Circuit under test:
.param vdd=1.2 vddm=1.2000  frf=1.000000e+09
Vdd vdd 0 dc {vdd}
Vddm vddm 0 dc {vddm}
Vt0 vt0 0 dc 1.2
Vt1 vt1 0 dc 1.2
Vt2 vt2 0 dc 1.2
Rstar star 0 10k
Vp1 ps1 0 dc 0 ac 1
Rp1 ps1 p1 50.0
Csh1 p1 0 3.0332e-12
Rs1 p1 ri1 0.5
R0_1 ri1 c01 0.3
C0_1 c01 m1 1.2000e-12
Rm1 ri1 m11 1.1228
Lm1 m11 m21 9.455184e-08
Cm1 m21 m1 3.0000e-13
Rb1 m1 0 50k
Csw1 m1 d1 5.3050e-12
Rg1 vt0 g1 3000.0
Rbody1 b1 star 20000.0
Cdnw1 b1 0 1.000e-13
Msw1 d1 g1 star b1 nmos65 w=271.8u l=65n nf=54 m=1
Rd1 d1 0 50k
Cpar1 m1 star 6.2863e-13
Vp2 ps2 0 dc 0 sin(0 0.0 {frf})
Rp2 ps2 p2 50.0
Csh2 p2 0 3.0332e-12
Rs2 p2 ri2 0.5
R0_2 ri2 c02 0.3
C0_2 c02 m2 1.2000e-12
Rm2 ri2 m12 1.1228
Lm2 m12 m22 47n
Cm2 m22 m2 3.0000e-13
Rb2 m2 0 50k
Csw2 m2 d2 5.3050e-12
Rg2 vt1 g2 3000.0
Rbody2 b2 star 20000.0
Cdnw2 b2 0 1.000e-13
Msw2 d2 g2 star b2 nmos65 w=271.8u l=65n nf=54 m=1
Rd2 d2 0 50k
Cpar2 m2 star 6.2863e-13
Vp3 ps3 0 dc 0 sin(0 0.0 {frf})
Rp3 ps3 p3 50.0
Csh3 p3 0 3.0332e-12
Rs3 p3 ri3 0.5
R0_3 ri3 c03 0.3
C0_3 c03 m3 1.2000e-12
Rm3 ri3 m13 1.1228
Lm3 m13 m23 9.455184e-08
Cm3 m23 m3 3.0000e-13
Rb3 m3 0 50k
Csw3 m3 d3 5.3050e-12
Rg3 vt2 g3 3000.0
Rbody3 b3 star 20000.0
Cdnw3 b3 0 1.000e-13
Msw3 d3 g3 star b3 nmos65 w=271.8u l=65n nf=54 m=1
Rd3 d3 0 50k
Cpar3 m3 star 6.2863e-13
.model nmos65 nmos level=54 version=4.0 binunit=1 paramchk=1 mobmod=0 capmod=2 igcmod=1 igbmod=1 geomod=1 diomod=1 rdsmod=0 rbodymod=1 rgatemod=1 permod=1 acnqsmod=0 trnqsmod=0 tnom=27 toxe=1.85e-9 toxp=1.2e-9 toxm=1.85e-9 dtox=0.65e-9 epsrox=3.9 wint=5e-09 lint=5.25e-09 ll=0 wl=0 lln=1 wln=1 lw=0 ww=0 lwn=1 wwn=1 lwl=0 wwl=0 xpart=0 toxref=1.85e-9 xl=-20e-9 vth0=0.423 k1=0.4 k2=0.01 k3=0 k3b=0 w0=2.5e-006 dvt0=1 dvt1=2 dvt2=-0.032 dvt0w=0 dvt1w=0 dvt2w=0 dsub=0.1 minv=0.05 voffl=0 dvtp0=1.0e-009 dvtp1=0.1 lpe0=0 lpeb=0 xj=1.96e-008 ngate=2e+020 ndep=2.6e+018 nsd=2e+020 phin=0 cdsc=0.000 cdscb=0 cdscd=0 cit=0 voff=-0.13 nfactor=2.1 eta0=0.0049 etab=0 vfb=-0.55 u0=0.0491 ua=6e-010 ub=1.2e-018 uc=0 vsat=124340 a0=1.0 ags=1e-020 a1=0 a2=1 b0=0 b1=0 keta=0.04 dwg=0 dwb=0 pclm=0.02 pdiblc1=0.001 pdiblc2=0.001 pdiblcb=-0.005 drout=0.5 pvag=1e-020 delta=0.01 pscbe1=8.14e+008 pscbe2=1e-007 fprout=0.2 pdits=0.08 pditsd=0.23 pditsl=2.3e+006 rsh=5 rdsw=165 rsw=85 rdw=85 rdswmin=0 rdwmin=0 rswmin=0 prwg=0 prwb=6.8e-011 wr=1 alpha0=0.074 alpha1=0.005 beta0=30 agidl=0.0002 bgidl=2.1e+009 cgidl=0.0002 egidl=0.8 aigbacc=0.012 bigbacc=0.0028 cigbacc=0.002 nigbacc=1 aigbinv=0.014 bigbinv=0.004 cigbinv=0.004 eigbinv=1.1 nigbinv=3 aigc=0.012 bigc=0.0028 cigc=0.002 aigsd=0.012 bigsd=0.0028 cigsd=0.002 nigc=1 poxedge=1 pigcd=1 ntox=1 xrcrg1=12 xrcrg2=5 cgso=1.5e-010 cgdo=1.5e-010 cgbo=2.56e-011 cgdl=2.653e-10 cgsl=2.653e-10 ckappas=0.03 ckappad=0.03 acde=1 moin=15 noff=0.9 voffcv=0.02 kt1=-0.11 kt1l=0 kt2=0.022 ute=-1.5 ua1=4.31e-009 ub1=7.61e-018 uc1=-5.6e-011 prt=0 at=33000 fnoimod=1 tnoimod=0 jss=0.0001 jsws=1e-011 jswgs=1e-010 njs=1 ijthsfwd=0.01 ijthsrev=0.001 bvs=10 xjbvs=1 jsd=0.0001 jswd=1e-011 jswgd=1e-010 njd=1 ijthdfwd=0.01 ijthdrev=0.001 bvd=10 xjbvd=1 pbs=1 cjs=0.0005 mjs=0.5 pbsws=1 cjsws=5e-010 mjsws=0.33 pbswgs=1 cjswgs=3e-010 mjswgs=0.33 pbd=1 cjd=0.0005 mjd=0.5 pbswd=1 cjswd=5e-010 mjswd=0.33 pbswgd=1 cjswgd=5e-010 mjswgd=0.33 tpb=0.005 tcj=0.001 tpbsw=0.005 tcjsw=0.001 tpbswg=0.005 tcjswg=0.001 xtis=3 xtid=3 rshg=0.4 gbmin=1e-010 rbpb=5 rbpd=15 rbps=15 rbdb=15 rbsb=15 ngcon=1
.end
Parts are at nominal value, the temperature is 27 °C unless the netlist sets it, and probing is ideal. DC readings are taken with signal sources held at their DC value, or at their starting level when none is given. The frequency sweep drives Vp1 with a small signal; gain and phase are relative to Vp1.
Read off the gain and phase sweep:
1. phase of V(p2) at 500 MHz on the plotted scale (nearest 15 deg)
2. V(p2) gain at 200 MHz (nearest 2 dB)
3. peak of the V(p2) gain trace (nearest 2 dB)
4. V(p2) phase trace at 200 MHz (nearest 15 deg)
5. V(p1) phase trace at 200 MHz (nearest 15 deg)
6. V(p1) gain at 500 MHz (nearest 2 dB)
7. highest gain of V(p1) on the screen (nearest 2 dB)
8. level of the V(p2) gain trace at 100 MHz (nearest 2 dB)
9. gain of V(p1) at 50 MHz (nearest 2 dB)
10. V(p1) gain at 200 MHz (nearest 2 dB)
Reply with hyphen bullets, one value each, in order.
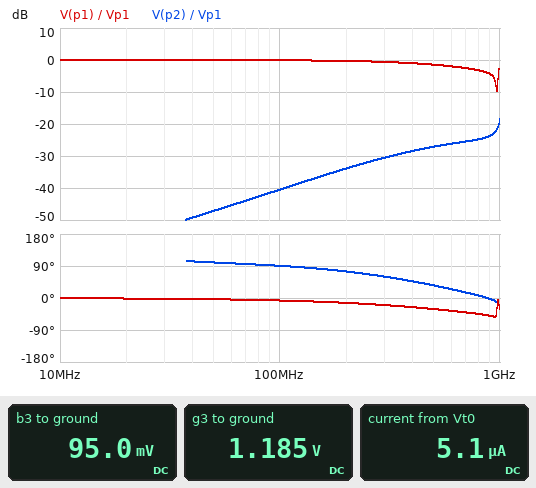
- 30 deg
- -34 dB
- -18 dB
- 75 deg
- -15 deg
- -2 dB
- 0 dB
- -40 dB
- 0 dB
- 0 dB
